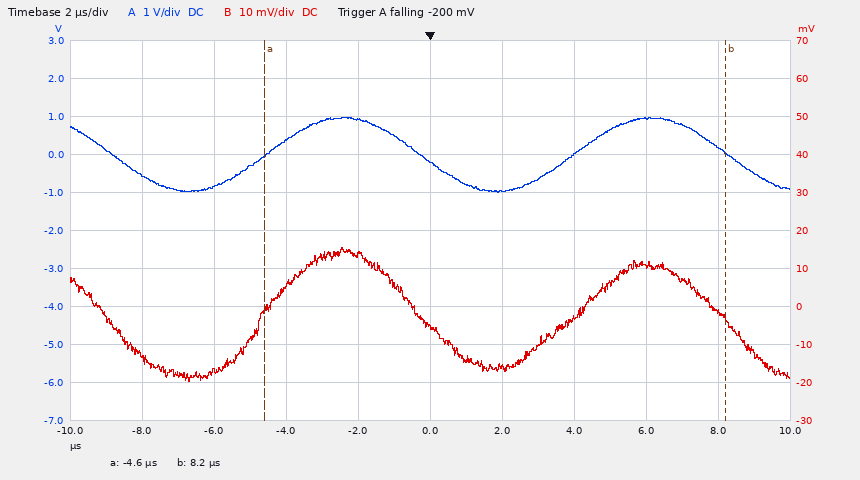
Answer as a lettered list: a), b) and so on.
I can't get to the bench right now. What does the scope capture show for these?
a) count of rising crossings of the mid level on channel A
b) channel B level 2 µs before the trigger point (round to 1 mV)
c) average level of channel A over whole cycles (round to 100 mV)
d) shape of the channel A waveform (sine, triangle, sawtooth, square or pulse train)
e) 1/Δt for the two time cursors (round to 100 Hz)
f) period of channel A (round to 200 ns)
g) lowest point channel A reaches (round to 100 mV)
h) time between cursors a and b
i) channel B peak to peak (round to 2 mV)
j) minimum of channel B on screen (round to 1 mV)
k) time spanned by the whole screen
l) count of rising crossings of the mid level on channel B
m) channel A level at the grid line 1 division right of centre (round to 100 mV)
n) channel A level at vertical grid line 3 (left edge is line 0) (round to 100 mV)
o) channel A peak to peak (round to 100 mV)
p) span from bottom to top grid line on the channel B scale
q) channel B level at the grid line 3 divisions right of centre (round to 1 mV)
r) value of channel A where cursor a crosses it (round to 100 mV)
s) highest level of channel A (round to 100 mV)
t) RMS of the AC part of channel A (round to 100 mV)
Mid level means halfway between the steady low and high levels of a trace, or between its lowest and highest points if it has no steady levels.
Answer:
a) 2
b) 14 mV
c) 0.0 V
d) sine
e) 78.1 kHz
f) 8.6 µs
g) -1.0 V
h) 12.8 µs
i) 36 mV
j) -20 mV
k) 20 µs
l) 2
m) -1.0 V
n) 400 mV
o) 2.0 V
p) 100 mV
q) 11 mV
r) 0.0 V
s) 1.0 V
t) 700 mV
